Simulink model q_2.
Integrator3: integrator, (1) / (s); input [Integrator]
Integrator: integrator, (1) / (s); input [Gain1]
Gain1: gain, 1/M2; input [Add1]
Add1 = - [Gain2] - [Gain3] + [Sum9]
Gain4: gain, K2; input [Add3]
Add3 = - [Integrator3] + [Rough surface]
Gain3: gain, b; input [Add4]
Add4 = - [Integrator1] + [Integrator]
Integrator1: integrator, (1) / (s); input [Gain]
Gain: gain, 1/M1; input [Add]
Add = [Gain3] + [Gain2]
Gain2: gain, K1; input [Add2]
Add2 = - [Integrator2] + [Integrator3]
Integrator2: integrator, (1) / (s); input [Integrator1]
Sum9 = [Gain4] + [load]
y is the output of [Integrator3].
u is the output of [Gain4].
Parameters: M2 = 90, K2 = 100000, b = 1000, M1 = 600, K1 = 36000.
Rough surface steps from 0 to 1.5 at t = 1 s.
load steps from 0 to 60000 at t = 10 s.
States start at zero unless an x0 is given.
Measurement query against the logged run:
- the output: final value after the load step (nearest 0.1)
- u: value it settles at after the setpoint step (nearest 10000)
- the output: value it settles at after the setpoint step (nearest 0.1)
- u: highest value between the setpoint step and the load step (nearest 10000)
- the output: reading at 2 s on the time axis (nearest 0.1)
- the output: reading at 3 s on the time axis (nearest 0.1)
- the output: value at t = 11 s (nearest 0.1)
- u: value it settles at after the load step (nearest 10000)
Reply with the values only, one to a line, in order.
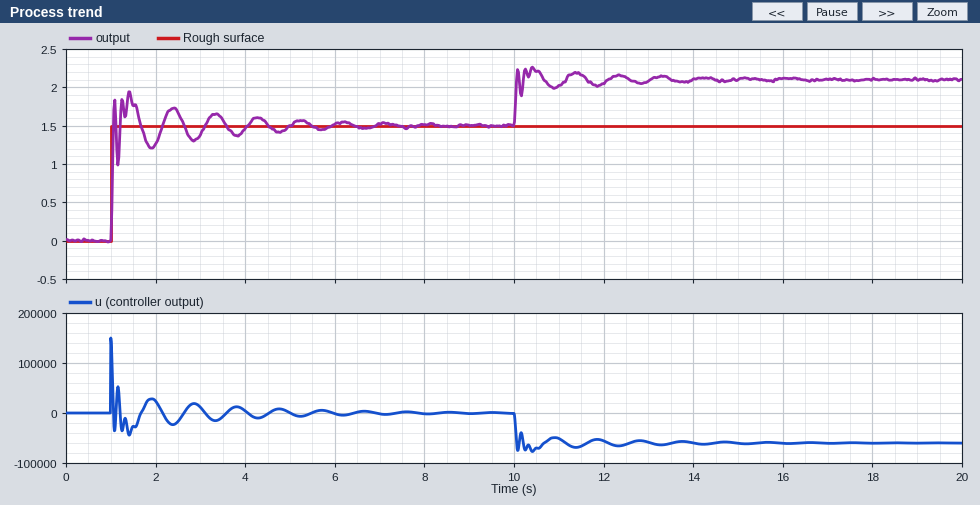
2.1
0
1.5
150000
1.3
1.4
2.0
-60000
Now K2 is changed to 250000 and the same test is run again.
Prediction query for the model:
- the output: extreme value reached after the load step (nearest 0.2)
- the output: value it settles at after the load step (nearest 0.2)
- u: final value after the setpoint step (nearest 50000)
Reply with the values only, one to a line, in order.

1.8
1.8
0
